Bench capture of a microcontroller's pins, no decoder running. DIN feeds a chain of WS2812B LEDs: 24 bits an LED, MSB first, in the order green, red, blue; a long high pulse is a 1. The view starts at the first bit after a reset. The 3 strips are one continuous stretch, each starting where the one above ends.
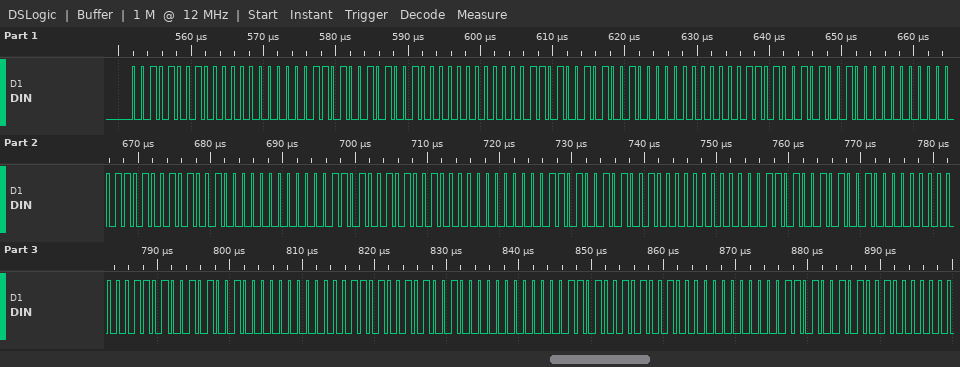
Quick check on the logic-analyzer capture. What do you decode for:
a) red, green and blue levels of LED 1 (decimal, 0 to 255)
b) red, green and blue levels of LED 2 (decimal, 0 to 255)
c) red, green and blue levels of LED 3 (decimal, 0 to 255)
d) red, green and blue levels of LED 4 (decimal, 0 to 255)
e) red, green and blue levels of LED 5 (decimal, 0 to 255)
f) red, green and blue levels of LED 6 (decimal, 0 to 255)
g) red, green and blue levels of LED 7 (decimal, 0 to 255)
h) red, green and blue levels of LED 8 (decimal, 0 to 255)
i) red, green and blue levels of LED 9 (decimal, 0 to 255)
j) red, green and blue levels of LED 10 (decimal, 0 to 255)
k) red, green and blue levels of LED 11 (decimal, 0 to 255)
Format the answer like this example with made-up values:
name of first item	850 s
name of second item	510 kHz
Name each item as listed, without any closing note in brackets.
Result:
red, green and blue levels of LED 1	0, 41, 13
red, green and blue levels of LED 2	0, 41, 13
red, green and blue levels of LED 3	0, 41, 13
red, green and blue levels of LED 4	0, 41, 13
red, green and blue levels of LED 5	0, 41, 13
red, green and blue levels of LED 6	0, 41, 13
red, green and blue levels of LED 7	0, 41, 13
red, green and blue levels of LED 8	0, 41, 13
red, green and blue levels of LED 9	0, 41, 13
red, green and blue levels of LED 10	0, 41, 13
red, green and blue levels of LED 11	0, 41, 13
